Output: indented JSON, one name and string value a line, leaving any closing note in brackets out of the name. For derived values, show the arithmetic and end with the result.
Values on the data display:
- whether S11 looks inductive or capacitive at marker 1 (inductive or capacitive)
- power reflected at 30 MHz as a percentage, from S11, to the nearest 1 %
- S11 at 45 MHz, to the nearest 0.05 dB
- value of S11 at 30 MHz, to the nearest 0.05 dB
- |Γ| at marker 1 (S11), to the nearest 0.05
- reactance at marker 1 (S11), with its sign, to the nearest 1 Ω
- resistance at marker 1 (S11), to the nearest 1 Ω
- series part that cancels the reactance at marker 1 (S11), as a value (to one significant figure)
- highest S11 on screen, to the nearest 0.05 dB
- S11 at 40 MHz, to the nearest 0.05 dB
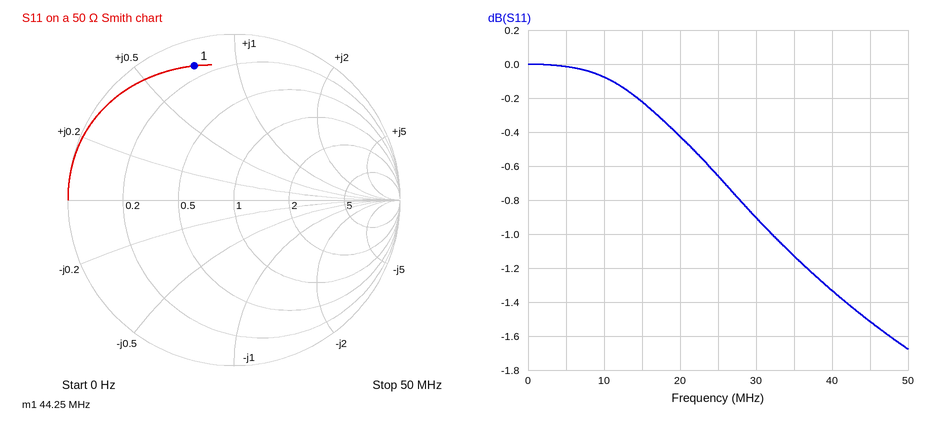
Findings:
{
  "whether S11 looks inductive or capacitive at marker 1": "inductive",
  "power reflected at 30 MHz as a percentage, from S11, to the nearest 1 %": "10^(-0.9/10) ≈ 81 %",
  "S11 at 45 MHz, to the nearest 0.05 dB": "-1.50 dB",
  "value of S11 at 30 MHz, to the nearest 0.05 dB": "-0.90 dB",
  "|Γ| at marker 1 (S11), to the nearest 0.05": "0.85",
  "reactance at marker 1 (S11), with its sign, to the nearest 1 Ω": "+37 Ω",
  "resistance at marker 1 (S11), to the nearest 1 Ω": "7 Ω",
  "series part that cancels the reactance at marker 1 (S11), as a value": "C = 1/(2π × 44.25 MHz × 37 Ω) ≈ 97.2 pF, so 100 pF to one significant figure",
  "highest S11 on screen, to the nearest 0.05 dB": "0.00 dB",
  "S11 at 40 MHz, to the nearest 0.05 dB": "-1.35 dB"
}
